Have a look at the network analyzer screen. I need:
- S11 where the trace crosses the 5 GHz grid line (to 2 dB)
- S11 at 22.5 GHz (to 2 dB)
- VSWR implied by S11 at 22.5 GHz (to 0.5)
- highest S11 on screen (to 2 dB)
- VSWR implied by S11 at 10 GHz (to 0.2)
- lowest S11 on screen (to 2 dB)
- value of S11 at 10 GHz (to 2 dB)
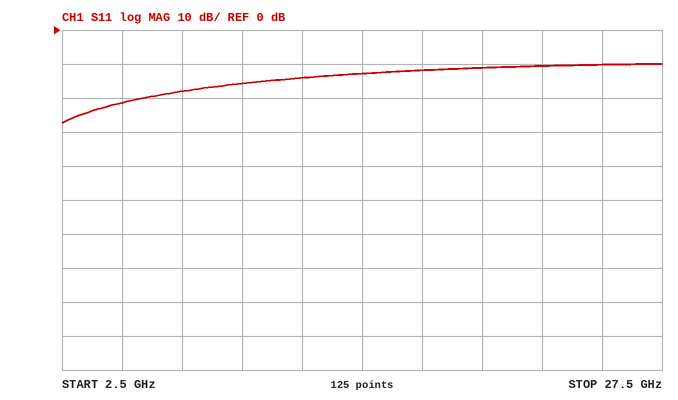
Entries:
-22 dB
-10 dB
2.0
-10 dB
1.4
-28 dB
-16 dB
